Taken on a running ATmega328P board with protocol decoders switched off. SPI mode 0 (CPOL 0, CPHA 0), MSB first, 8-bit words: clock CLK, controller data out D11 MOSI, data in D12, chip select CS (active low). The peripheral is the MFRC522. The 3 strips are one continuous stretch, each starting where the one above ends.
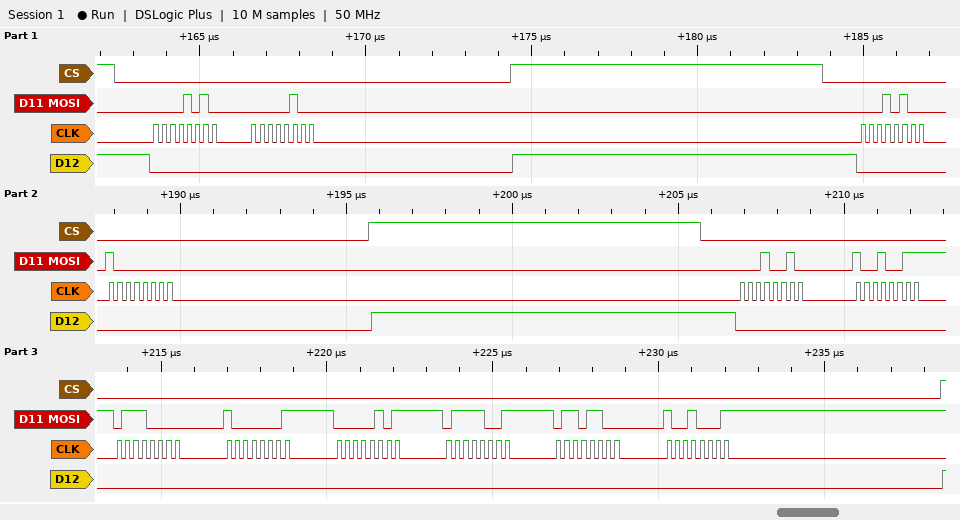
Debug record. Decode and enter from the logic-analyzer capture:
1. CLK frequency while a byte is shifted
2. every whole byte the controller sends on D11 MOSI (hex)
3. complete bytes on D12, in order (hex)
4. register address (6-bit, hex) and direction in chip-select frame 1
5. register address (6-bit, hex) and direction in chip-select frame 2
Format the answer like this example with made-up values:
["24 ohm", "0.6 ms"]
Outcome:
["4 MHz", "0A 04 14 80 12 93 70 81 05 79 6C 91", "00 00 00 00 00 00 00 00 00 00 00 00", "0x05 write", "0x0A write"]
